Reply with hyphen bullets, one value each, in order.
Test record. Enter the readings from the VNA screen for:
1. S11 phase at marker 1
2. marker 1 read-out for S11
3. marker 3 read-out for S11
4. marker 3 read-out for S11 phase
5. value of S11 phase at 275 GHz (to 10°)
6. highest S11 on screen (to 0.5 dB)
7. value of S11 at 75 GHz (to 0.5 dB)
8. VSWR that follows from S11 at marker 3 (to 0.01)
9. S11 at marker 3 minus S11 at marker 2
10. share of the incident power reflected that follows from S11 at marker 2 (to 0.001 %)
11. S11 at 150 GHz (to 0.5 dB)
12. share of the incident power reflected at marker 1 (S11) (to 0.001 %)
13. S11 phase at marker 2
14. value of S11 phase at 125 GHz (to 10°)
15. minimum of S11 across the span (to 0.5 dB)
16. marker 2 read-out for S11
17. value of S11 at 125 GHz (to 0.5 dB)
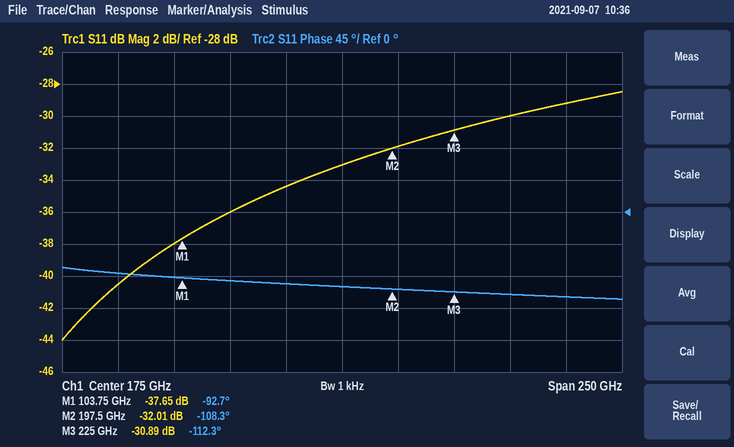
- -92.7°
- -37.65 dB
- -30.89 dB
- -112.3°
- -120°
- -28.5 dB
- -40.5 dB
- 1.06
- 1.12 dB
- 0.063 %
- -34.5 dB
- 0.017 %
- -108.3°
- -100°
- -44.0 dB
- -32.01 dB
- -36.0 dB
